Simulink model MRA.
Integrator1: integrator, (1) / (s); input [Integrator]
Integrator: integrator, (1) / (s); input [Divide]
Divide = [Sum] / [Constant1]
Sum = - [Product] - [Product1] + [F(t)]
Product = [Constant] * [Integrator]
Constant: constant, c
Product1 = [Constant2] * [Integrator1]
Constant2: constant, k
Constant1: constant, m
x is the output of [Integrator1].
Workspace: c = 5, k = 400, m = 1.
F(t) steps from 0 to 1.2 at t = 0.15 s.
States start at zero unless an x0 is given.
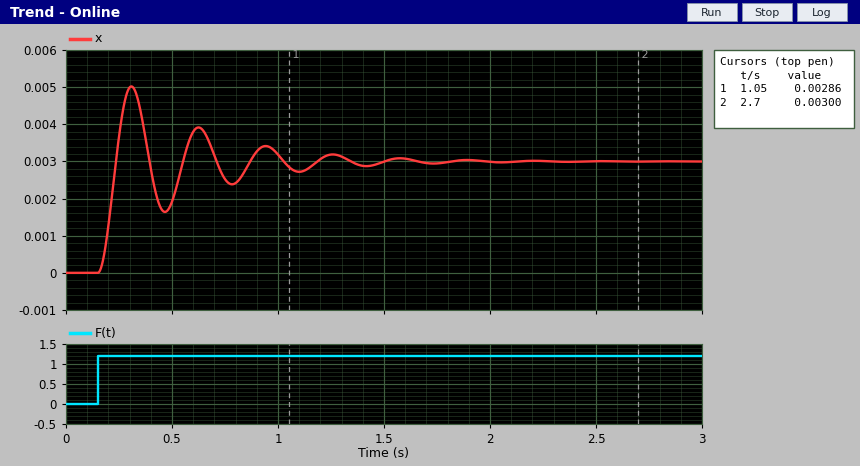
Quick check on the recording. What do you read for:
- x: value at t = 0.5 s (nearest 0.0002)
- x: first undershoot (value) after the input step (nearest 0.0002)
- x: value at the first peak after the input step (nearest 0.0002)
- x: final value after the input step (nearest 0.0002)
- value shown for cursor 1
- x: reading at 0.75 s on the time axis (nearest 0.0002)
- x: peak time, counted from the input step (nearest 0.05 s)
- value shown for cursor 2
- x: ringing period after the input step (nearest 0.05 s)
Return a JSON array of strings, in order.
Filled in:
["0.0020", "0.0016", "0.0050", "0.0030", "0.00286", "0.0026", "0.15 s", "0.00300", "0.30 s"]
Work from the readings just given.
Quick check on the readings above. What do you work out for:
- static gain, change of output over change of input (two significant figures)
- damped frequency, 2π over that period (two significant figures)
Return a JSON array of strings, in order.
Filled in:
["0.0025", "21 rad/s"]
